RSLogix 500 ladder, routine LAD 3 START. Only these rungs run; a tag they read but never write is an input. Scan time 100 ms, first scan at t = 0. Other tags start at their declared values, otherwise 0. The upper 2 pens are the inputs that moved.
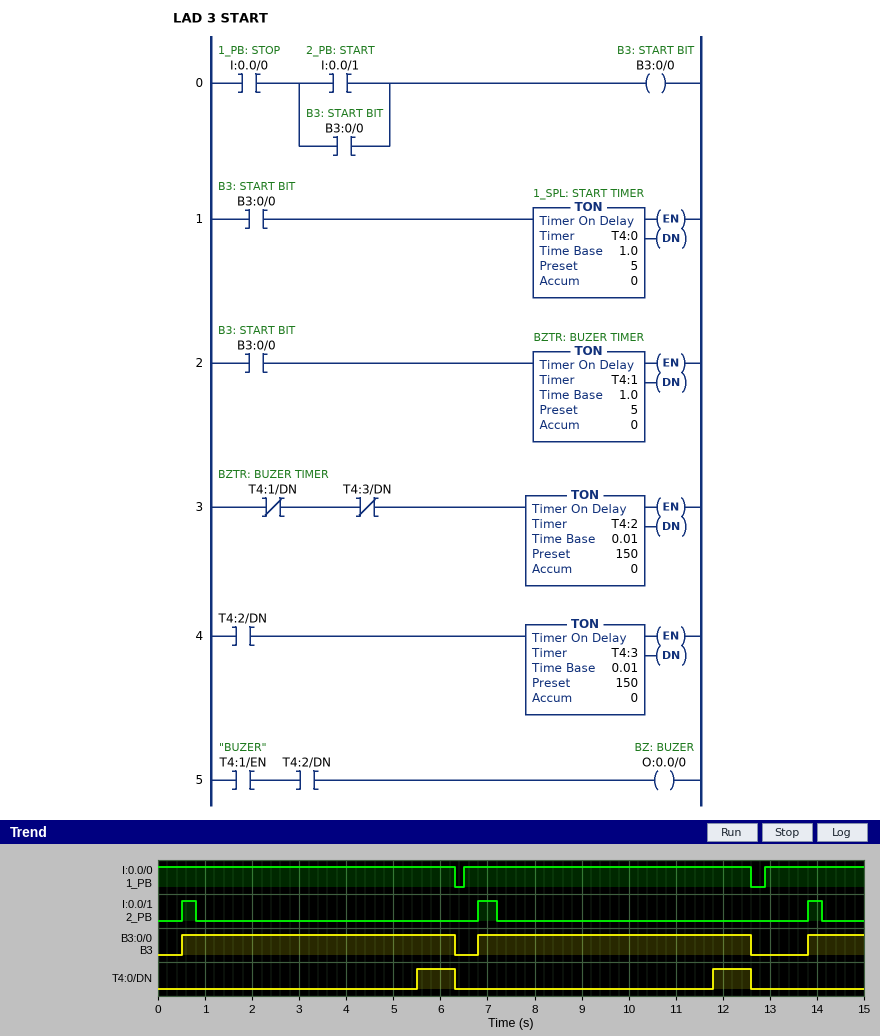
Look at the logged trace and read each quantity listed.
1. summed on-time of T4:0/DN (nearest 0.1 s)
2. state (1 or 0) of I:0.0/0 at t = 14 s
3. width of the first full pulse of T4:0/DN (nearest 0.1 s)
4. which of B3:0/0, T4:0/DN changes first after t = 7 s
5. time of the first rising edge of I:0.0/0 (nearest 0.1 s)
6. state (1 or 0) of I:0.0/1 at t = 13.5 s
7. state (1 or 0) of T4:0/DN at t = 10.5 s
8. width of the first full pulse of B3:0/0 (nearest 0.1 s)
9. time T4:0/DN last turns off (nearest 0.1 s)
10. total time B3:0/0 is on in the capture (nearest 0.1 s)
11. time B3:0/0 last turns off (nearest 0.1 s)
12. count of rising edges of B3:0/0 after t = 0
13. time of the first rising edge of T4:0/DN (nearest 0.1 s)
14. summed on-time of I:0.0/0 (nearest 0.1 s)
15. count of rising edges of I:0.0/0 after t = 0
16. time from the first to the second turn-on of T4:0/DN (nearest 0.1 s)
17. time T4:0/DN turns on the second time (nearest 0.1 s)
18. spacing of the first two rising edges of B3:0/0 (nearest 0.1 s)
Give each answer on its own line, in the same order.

1.6 s
1
0.8 s
T4:0/DN
6.5 s
0
0
5.8 s
12.6 s
12.8 s
12.6 s
3
5.5 s
14.5 s
2
6.3 s
11.8 s
6.3 s
